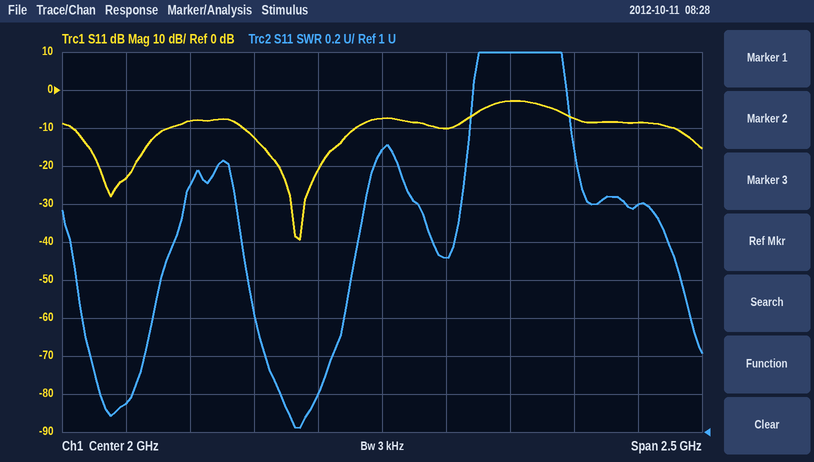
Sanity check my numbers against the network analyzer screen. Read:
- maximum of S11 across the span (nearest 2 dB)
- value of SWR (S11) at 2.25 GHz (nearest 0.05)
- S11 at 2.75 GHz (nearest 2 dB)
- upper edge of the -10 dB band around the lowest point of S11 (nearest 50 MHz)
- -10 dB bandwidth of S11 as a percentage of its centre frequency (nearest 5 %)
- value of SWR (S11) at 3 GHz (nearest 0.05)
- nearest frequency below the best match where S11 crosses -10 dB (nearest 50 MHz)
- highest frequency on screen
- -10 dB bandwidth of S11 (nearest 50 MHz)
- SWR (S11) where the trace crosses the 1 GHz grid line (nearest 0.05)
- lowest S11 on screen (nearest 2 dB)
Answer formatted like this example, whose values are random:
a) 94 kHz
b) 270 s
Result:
a) -2 dB
b) 1.90
c) -8 dB
d) 1.90 GHz
e) 25 %
f) 2.20
g) 1.45 GHz
h) 3.25 GHz
i) 450 MHz
j) 1.15
k) -40 dB
